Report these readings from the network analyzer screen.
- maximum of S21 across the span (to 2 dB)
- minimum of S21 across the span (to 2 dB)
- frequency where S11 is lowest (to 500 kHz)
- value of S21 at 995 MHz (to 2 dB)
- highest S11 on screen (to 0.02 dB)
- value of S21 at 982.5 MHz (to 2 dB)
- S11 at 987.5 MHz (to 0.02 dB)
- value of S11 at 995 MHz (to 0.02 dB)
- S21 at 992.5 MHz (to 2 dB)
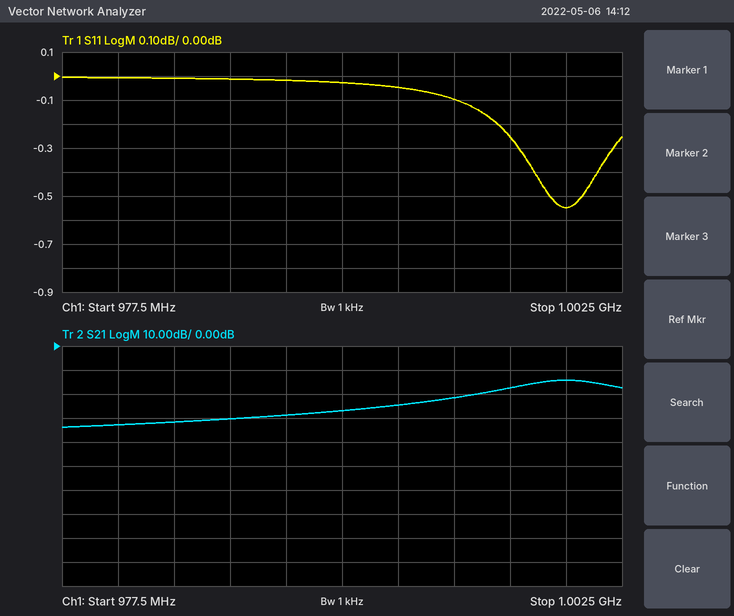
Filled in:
-14 dB
-34 dB
1.0000 GHz
-22 dB
0.00 dB
-32 dB
-0.02 dB
-0.10 dB
-24 dB
